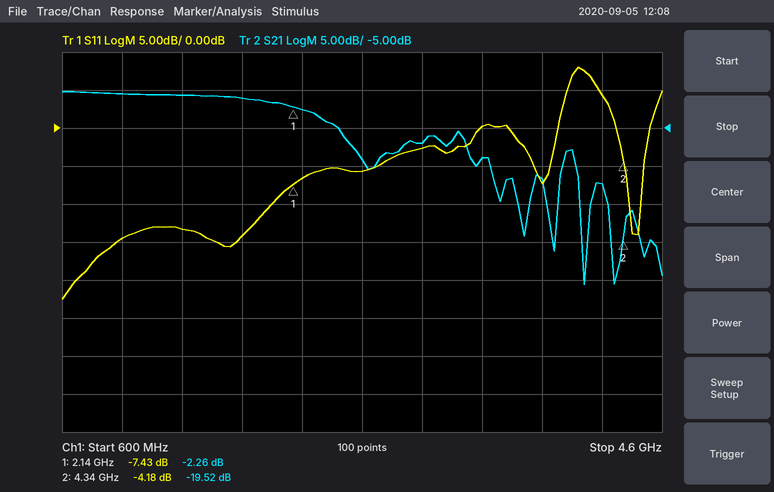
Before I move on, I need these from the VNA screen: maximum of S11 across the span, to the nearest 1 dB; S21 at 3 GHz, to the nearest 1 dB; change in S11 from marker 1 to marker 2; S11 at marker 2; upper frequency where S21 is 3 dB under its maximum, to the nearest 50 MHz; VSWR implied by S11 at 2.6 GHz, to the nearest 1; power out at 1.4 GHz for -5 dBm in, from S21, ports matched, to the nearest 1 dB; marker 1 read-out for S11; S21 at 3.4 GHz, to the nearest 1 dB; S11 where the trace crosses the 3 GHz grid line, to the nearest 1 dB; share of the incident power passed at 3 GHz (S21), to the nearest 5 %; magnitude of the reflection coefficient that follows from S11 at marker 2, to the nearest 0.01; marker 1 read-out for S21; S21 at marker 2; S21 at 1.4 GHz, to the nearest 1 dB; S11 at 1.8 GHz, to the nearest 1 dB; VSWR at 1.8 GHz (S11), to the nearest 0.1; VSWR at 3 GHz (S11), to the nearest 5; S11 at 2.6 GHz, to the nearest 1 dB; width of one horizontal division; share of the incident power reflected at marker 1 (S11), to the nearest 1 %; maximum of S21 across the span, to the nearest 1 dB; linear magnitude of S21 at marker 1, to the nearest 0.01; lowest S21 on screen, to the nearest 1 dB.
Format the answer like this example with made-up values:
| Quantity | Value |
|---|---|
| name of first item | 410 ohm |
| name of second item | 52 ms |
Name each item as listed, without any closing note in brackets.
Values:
| Quantity | Value |
|---|---|
| maximum of S11 across the span, to the nearest 1 dB | 8 dB |
| S21 at 3 GHz, to the nearest 1 dB | -7 dB |
| change in S11 from marker 1 to marker 2 | 3.25 dB |
| S11 at marker 2 | -4.18 dB |
| upper frequency where S21 is 3 dB under its maximum, to the nearest 50 MHz | 2.30 GHz |
| VSWR implied by S11 at 2.6 GHz, to the nearest 1 | 3 |
| power out at 1.4 GHz for -5 dBm in, from S21, ports matched, to the nearest 1 dB | -6 dBm |
| marker 1 read-out for S11 | -7.43 dB |
| S21 at 3.4 GHz, to the nearest 1 dB | -9 dB |
| S11 where the trace crosses the 3 GHz grid line, to the nearest 1 dB | -3 dB |
| share of the incident power passed at 3 GHz (S21), to the nearest 5 % | 20 % |
| magnitude of the reflection coefficient that follows from S11 at marker 2, to the nearest 0.01 | 0.62 |
| marker 1 read-out for S21 | -2.26 dB |
| S21 at marker 2 | -19.52 dB |
| S21 at 1.4 GHz, to the nearest 1 dB | -1 dB |
| S11 at 1.8 GHz, to the nearest 1 dB | -14 dB |
| VSWR at 1.8 GHz (S11), to the nearest 0.1 | 1.5 |
| VSWR at 3 GHz (S11), to the nearest 5 | 5 |
| S11 at 2.6 GHz, to the nearest 1 dB | -6 dB |
| width of one horizontal division | 400 MHz |
| share of the incident power reflected at marker 1 (S11), to the nearest 1 % | 18 % |
| maximum of S21 across the span, to the nearest 1 dB | 0 dB |
| linear magnitude of S21 at marker 1, to the nearest 0.01 | 0.77 |
| lowest S21 on screen, to the nearest 1 dB | -26 dB |
